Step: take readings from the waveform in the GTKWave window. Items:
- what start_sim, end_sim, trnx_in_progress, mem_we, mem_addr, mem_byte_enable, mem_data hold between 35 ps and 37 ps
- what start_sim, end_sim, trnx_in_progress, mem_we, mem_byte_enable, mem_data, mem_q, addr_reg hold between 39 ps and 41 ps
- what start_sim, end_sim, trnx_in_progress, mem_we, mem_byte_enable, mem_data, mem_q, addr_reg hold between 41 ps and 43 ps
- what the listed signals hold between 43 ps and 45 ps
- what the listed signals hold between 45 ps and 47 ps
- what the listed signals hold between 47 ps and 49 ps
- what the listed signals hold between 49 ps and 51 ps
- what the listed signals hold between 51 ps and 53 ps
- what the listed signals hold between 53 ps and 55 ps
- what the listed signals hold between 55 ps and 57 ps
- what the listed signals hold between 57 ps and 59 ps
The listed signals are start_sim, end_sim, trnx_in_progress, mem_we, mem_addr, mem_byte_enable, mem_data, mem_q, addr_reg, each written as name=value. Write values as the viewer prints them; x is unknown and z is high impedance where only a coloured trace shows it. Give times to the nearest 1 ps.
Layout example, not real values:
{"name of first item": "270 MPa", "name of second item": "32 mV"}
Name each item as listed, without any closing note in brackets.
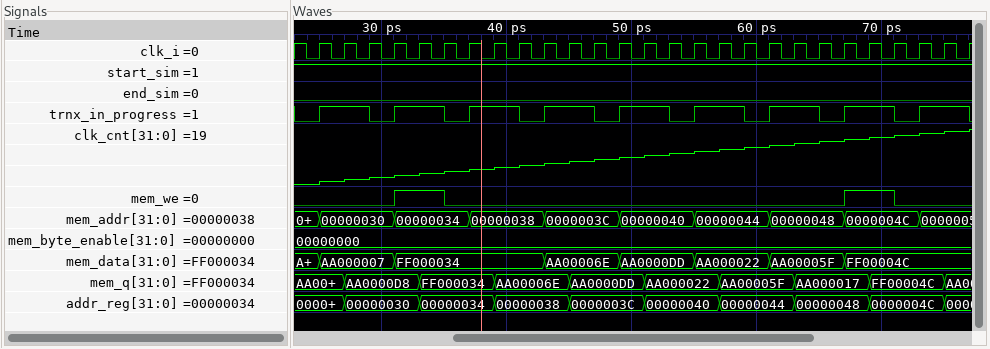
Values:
{"what start_sim, end_sim, trnx_in_progress, mem_we, mem_addr, mem_byte_enable, mem_data hold between 35 ps and 37 ps": "start_sim=1, end_sim=0, trnx_in_progress=0, mem_we=0, mem_addr=00000034, mem_byte_enable=00000000, mem_data=FF000034", "what start_sim, end_sim, trnx_in_progress, mem_we, mem_byte_enable, mem_data, mem_q, addr_reg hold between 39 ps and 41 ps": "start_sim=1, end_sim=0, trnx_in_progress=1, mem_we=0, mem_byte_enable=00000000, mem_data=FF000034, mem_q=AA00006E, addr_reg=00000038", "what start_sim, end_sim, trnx_in_progress, mem_we, mem_byte_enable, mem_data, mem_q, addr_reg hold between 41 ps and 43 ps": "start_sim=1, end_sim=0, trnx_in_progress=0, mem_we=0, mem_byte_enable=00000000, mem_data=FF000034, mem_q=AA00006E, addr_reg=00000038", "what the listed signals hold between 43 ps and 45 ps": "start_sim=1, end_sim=0, trnx_in_progress=1, mem_we=0, mem_addr=0000003C, mem_byte_enable=00000000, mem_data=AA00006E, mem_q=AA00006E, addr_reg=00000038", "what the listed signals hold between 45 ps and 47 ps": "start_sim=1, end_sim=0, trnx_in_progress=1, mem_we=0, mem_addr=0000003C, mem_byte_enable=00000000, mem_data=AA00006E, mem_q=AA0000DD, addr_reg=0000003C", "what the listed signals hold between 47 ps and 49 ps": "start_sim=1, end_sim=0, trnx_in_progress=0, mem_we=0, mem_addr=0000003C, mem_byte_enable=00000000, mem_data=AA00006E, mem_q=AA0000DD, addr_reg=0000003C", "what the listed signals hold between 49 ps and 51 ps": "start_sim=1, end_sim=0, trnx_in_progress=1, mem_we=0, mem_addr=00000040, mem_byte_enable=00000000, mem_data=AA0000DD, mem_q=AA0000DD, addr_reg=0000003C", "what the listed signals hold between 51 ps and 53 ps": "start_sim=1, end_sim=0, trnx_in_progress=1, mem_we=0, mem_addr=00000040, mem_byte_enable=00000000, mem_data=AA0000DD, mem_q=AA000022, addr_reg=00000040", "what the listed signals hold between 53 ps and 55 ps": "start_sim=1, end_sim=0, trnx_in_progress=0, mem_we=0, mem_addr=00000040, mem_byte_enable=00000000, mem_data=AA0000DD, mem_q=AA000022, addr_reg=00000040", "what the listed signals hold between 55 ps and 57 ps": "start_sim=1, end_sim=0, trnx_in_progress=1, mem_we=0, mem_addr=00000044, mem_byte_enable=00000000, mem_data=AA000022, mem_q=AA000022, addr_reg=00000040", "what the listed signals hold between 57 ps and 59 ps": "start_sim=1, end_sim=0, trnx_in_progress=1, mem_we=0, mem_addr=00000044, mem_byte_enable=00000000, mem_data=AA000022, mem_q=AA00005F, addr_reg=00000044"}
